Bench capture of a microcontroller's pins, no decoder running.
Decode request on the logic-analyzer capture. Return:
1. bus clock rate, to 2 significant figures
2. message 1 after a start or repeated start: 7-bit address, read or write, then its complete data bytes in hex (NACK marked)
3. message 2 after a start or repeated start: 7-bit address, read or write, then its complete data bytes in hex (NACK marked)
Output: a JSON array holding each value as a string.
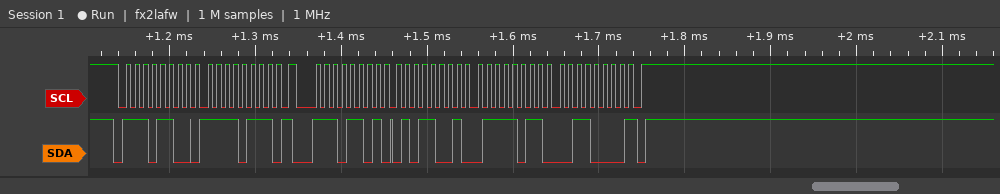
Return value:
["100 kHz", "0x76 write: F7", "0x76 read: 59 7B 30 NACK"]
